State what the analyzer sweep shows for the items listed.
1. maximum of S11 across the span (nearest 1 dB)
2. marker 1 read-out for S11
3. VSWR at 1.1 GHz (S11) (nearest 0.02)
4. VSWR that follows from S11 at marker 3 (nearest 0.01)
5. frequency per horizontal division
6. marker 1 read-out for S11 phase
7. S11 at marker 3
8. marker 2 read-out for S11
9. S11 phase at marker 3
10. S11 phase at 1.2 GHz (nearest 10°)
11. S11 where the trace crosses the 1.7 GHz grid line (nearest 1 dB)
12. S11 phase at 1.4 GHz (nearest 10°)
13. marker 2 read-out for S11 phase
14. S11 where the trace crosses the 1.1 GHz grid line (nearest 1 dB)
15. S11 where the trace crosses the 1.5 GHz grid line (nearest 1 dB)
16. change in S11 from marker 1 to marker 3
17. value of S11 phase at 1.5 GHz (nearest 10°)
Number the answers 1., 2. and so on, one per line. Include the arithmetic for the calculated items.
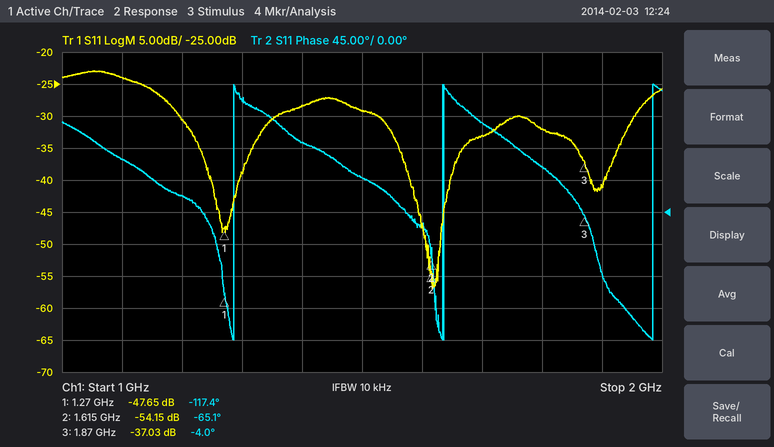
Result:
1. -23 dB
2. -47.65 dB
3. |Γ| = 10^(-24/20) = 0.0631; VSWR = (1 + 0.0631)/(1 − 0.0631) ≈ 1.13, so 1.14 to the nearest 0.02
4. (1 + 0.0141)/(1 − 0.0141) ≈ 1.03
5. 100 MHz
6. -117.4°
7. -37.03 dB
8. -54.15 dB
9. -4.0°
10. 20°
11. -33 dB
12. 100°
13. -65.1°
14. -24 dB
15. -29 dB
16. -37.03 − (-47.65) = 10.62 dB
17. 50°
